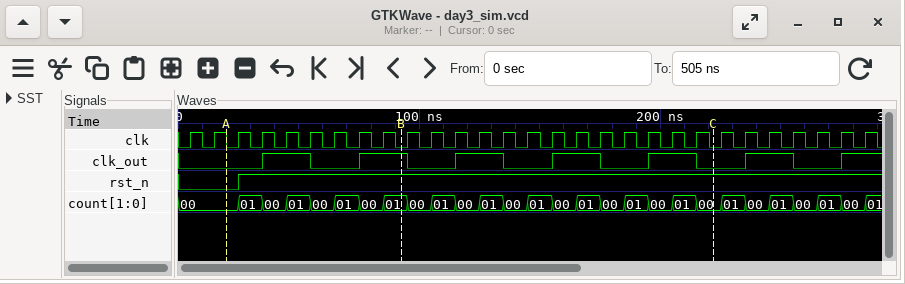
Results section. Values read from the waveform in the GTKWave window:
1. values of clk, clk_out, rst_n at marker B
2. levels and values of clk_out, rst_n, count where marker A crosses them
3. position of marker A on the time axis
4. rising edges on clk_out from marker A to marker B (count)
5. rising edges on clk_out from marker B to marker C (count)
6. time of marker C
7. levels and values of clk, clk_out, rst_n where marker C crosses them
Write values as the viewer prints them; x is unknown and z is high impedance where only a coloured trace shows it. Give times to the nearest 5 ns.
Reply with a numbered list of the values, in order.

1. clk=0, clk_out=1, rst_n=1
2. clk_out=0, rst_n=0, count=00
3. 20 ns
4. 2
5. 3
6. 220 ns
7. clk=0, clk_out=0, rst_n=1
